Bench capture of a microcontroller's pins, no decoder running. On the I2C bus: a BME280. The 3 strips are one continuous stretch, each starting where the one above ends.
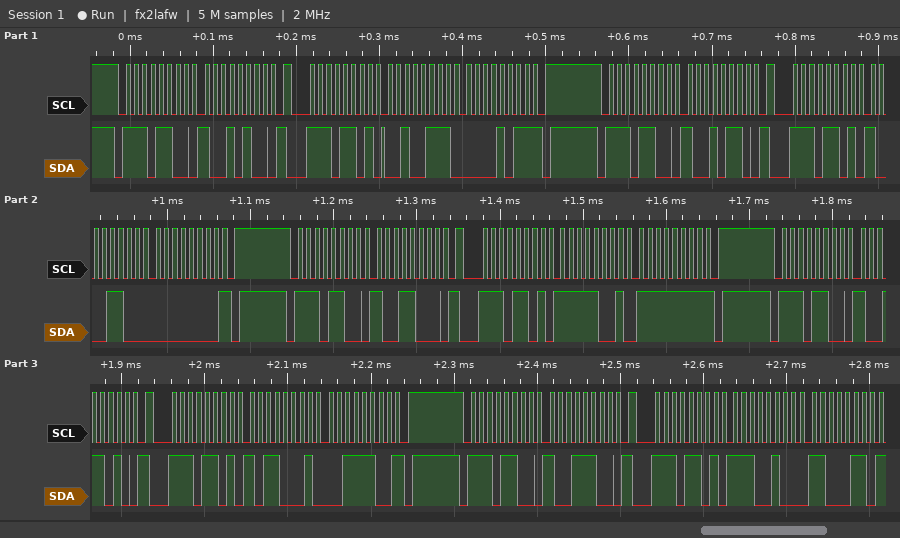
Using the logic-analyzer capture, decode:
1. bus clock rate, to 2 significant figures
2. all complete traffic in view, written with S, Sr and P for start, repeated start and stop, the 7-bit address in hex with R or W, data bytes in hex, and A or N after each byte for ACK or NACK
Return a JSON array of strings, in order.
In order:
["100 kHz", "S 76W A 94 A Sr 76R A 27 A 0B N P S 76W A 96 A Sr 76R A 8C A 00 N P S 76W A 98 A Sr 76R A F9 A FF N P S 76W A 9A A Sr 76R A B1 A 3C N P S 76W A 9C A Sr 76R A E4 A C6 N"]
